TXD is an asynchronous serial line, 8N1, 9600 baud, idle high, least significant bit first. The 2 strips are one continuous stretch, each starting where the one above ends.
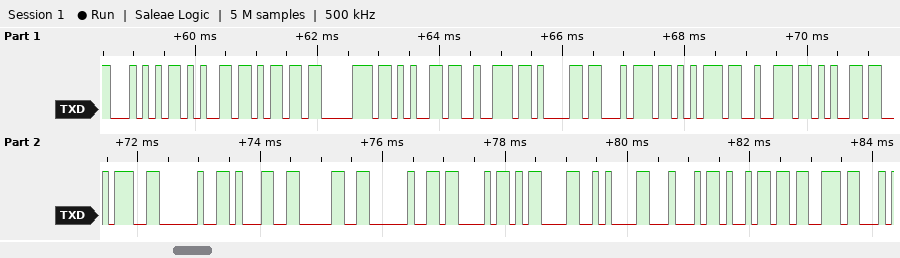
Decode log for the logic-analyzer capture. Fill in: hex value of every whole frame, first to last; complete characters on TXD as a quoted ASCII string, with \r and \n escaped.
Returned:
54 65 6D 70 65 72 61 74 75 72 65 3A 20 31 30 20 43 0D 0A 44 69 73
"Temperature: 10 C\r\nDis"
